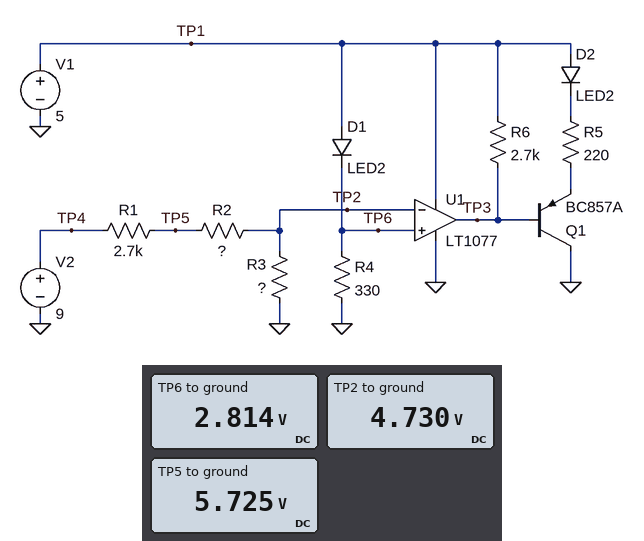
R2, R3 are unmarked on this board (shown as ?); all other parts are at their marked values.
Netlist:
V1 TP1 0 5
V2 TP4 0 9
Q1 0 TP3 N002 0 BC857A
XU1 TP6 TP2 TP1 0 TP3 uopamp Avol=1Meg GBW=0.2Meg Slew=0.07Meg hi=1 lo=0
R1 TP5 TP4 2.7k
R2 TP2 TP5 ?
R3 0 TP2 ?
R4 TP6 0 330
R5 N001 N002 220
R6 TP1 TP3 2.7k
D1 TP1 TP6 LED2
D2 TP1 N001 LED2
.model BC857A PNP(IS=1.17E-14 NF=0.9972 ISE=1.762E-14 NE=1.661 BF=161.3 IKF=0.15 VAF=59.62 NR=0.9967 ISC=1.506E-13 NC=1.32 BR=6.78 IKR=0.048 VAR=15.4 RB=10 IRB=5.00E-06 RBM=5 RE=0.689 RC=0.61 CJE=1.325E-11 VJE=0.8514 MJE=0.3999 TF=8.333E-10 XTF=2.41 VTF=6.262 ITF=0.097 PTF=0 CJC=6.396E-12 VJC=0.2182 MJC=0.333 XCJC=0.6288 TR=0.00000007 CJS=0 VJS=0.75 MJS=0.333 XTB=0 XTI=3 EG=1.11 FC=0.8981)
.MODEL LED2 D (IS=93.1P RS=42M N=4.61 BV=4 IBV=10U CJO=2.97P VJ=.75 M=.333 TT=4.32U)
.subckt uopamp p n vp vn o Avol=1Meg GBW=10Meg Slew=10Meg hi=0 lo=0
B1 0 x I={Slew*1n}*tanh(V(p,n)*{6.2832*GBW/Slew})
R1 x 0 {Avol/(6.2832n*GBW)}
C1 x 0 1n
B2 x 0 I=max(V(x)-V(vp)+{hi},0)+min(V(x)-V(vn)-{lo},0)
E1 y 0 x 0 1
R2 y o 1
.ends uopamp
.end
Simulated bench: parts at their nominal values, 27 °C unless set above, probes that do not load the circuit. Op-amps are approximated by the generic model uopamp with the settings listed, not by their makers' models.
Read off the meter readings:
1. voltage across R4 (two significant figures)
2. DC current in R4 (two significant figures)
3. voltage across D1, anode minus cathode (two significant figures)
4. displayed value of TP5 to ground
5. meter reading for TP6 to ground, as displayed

2.8 V
8.5 mA
2.2 V
5.725 V
2.814 V
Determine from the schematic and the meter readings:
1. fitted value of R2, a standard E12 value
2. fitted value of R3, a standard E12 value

820 Ω
3.9 kΩ
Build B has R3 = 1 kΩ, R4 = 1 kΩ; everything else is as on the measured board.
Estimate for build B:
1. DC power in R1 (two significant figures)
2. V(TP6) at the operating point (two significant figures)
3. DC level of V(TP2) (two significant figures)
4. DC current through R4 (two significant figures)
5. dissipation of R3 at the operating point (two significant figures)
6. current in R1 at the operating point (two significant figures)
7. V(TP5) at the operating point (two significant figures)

11 mW
2.9 V
2.0 V
2.9 mA
4.0 mW
2.0 mA
3.6 V
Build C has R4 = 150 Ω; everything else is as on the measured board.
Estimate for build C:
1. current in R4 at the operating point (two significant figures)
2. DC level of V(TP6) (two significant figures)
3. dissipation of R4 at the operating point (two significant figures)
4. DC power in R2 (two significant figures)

18 mA
2.7 V
49 mW
1.2 mW
